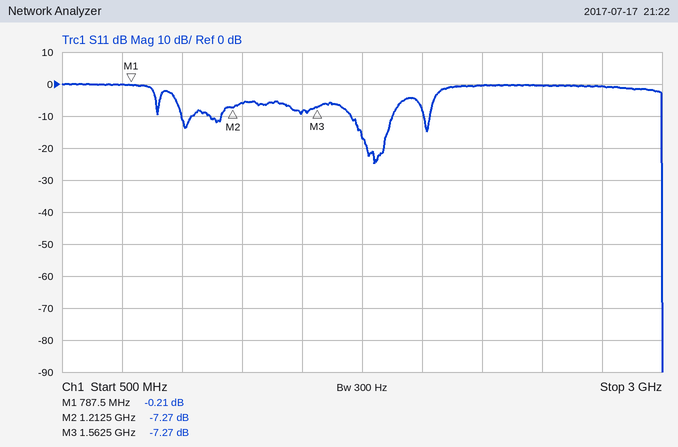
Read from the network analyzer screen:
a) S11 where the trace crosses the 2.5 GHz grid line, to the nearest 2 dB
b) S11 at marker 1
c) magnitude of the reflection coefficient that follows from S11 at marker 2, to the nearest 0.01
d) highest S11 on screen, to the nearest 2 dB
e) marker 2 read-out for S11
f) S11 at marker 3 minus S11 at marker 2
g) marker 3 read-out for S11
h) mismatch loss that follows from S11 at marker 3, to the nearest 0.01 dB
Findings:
0 dB
-0.21 dB
0.43
0 dB
-7.27 dB
0.00 dB
-7.27 dB
0.90 dB
